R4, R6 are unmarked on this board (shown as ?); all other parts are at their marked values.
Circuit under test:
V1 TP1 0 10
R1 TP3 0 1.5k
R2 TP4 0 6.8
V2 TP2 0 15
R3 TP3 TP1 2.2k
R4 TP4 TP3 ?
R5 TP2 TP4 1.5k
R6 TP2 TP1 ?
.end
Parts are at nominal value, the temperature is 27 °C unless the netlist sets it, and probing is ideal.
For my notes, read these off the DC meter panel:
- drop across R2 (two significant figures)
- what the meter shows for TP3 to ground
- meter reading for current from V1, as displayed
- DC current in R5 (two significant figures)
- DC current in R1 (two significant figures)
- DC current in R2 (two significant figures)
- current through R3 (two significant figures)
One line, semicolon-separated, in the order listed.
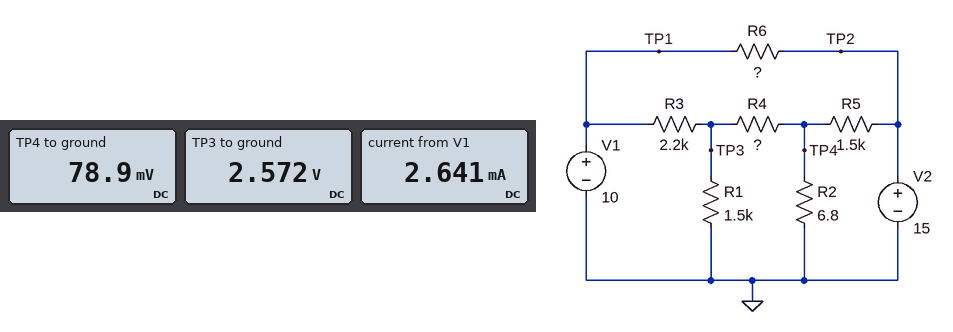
79 mV; 2.572 V; 2.641 mA; 9.9 mA; 1.7 mA; 12 mA; 3.4 mA
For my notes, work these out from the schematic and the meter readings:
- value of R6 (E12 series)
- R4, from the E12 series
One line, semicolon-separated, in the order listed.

6.8 kΩ; 1.5 kΩ
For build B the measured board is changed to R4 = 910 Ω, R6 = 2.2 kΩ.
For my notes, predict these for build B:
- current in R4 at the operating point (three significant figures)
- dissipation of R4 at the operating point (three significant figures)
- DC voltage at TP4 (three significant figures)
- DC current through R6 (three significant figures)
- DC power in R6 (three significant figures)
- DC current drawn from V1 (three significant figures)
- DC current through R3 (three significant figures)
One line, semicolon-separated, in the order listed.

2.20 mA; 4.42 mW; 82.6 mV; 2.27 mA; 11.4 mW; 1.32 mA; 3.60 mA
